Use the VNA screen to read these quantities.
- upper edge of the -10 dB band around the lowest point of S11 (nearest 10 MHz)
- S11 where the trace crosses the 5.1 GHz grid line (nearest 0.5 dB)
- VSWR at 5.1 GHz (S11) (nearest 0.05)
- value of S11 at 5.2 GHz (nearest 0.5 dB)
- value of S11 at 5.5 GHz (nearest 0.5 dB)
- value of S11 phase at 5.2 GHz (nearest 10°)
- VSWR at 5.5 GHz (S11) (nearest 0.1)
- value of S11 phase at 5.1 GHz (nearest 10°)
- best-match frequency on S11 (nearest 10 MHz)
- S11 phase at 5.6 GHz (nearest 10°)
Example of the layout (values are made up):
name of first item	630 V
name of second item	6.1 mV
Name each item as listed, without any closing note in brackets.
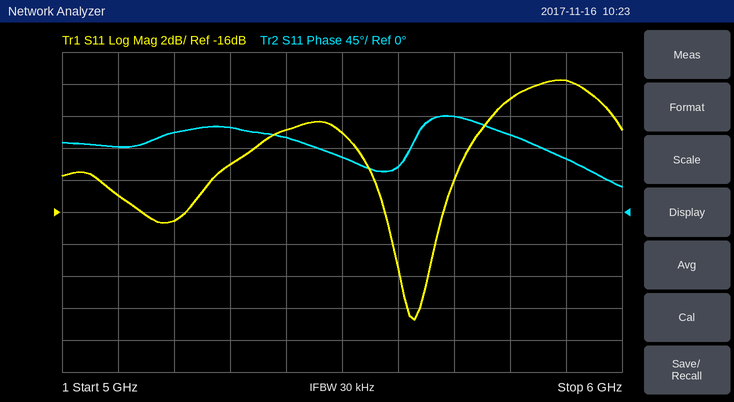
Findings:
upper edge of the -10 dB band around the lowest point of S11	5.77 GHz
S11 where the trace crosses the 5.1 GHz grid line	-15.0 dB
VSWR at 5.1 GHz (S11)	1.45
value of S11 at 5.2 GHz	-16.5 dB
value of S11 at 5.5 GHz	-11.0 dB
value of S11 phase at 5.2 GHz	110°
VSWR at 5.5 GHz (S11)	1.8
value of S11 phase at 5.1 GHz	90°
best-match frequency on S11	5.63 GHz
S11 phase at 5.6 GHz	60°
